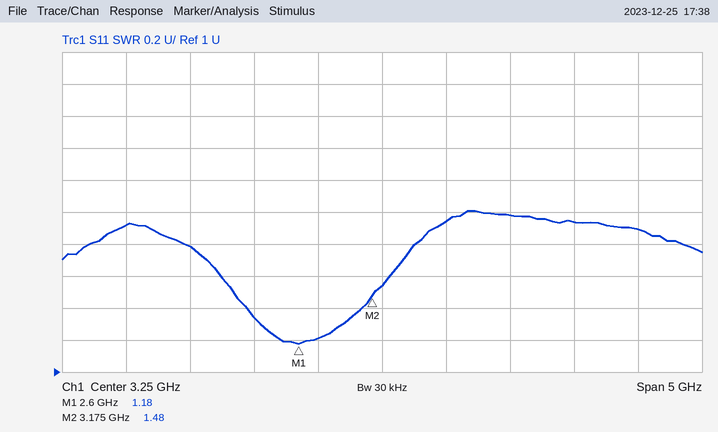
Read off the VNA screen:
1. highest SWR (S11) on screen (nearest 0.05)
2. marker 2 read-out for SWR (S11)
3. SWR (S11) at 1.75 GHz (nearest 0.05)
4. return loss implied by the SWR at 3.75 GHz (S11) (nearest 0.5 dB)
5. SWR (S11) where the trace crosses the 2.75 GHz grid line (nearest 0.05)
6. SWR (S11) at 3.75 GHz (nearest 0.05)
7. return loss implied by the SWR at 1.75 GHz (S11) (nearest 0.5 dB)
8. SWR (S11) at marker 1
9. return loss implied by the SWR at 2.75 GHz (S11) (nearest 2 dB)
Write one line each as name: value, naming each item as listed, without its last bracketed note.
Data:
highest SWR (S11) on screen: 2.00
marker 2 read-out for SWR: 1.48
SWR (S11) at 1.75 GHz: 1.80
return loss implied by the SWR at 3.75 GHz (S11): 10.0 dB
SWR (S11) where the trace crosses the 2.75 GHz grid line: 1.20
SWR (S11) at 3.75 GHz: 1.95
return loss implied by the SWR at 1.75 GHz (S11): 11.0 dB
SWR (S11) at marker 1: 1.18
return loss implied by the SWR at 2.75 GHz (S11): 20 dB
